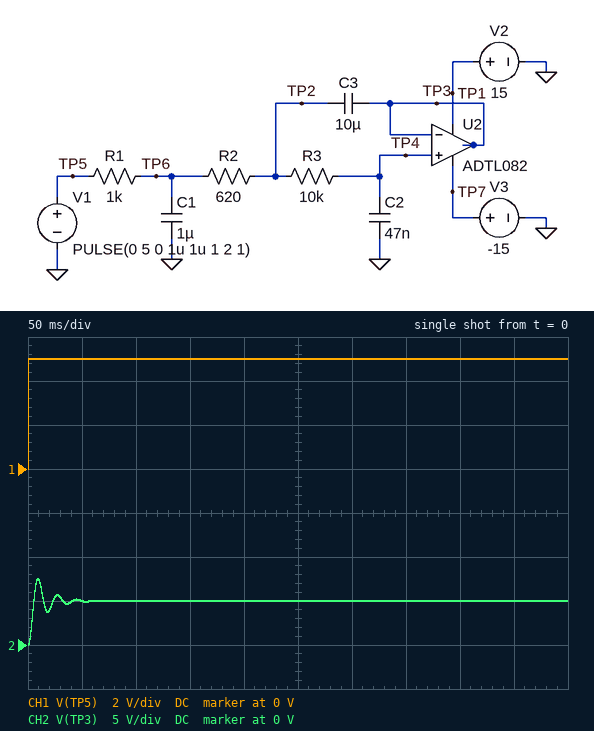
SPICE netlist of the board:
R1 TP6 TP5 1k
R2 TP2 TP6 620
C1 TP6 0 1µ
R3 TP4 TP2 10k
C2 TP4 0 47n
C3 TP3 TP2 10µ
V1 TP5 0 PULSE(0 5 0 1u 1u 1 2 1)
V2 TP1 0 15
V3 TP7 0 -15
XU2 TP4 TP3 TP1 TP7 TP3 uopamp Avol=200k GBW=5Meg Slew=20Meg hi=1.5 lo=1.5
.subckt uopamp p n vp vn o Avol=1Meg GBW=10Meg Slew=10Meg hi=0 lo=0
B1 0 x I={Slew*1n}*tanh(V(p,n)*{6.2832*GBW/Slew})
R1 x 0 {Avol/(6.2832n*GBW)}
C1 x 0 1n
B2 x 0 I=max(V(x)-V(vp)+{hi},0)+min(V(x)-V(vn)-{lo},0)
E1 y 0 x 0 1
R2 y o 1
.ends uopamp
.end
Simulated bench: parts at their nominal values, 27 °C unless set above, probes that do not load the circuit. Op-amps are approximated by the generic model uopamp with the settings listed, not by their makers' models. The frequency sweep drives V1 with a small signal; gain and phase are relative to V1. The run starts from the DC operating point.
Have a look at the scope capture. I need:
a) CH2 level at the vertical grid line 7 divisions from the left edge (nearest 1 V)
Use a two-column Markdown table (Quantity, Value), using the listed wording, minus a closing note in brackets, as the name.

| Quantity | Value |
|---|---|
| CH2 level at the vertical grid line 7 divisions from the left edge | 5 V |
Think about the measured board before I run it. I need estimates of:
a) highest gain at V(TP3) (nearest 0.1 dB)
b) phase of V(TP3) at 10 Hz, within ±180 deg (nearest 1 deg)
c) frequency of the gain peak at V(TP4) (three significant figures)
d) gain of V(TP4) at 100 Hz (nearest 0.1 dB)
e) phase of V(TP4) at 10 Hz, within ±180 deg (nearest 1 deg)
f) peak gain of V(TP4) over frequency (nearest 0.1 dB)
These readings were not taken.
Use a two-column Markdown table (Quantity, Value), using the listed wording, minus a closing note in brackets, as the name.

| Quantity | Value |
|---|---|
| highest gain at V(TP3) | 7.6 dB |
| phase of V(TP3) at 10 Hz, within ±180 deg | -6 deg |
| frequency of the gain peak at V(TP4) | 54.8 Hz |
| gain of V(TP4) at 100 Hz | -6.9 dB |
| phase of V(TP4) at 10 Hz, within ±180 deg | -6 deg |
| peak gain of V(TP4) over frequency | 7.6 dB |
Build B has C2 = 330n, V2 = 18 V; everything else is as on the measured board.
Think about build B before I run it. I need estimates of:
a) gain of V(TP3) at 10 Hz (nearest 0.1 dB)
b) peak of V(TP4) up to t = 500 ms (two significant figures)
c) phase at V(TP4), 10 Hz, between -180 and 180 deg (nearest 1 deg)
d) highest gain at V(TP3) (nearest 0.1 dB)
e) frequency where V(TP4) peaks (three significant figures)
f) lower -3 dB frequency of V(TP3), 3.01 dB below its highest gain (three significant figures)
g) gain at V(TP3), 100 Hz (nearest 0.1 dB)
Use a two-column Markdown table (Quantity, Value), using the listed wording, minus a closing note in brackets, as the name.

| Quantity | Value |
|---|---|
| gain of V(TP3) at 10 Hz | 1.6 dB |
| peak of V(TP4) up to t = 500 ms | 6.9 V |
| phase at V(TP4), 10 Hz, between -180 and 180 deg | -21 deg |
| highest gain at V(TP3) | 4.8 dB |
| frequency where V(TP4) peaks | 19.4 Hz |
| lower -3 dB frequency of V(TP3), 3.01 dB below its highest gain | 10.6 Hz |
| gain at V(TP3), 100 Hz | -26.7 dB |
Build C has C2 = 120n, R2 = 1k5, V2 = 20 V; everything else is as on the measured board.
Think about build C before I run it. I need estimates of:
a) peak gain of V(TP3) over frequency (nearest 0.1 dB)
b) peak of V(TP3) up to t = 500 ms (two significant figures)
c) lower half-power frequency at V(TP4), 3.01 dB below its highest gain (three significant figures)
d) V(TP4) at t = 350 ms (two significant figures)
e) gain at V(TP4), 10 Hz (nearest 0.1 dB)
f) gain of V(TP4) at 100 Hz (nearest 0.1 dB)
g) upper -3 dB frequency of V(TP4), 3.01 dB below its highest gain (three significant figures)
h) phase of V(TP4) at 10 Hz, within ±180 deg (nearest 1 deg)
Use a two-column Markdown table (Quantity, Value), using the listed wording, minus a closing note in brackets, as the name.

| Quantity | Value |
|---|---|
| peak gain of V(TP3) over frequency | 9.3 dB |
| peak of V(TP3) up to t = 500 ms | 7.9 V |
| lower half-power frequency at V(TP4), 3.01 dB below its highest gain | 22.4 Hz |
| V(TP4) at t = 350 ms | 5.0 V |
| gain at V(TP4), 10 Hz | 1.0 dB |
| gain of V(TP4) at 100 Hz | -21.4 dB |
| upper -3 dB frequency of V(TP4), 3.01 dB below its highest gain | 32.7 Hz |
| phase of V(TP4) at 10 Hz, within ±180 deg | -10 deg |
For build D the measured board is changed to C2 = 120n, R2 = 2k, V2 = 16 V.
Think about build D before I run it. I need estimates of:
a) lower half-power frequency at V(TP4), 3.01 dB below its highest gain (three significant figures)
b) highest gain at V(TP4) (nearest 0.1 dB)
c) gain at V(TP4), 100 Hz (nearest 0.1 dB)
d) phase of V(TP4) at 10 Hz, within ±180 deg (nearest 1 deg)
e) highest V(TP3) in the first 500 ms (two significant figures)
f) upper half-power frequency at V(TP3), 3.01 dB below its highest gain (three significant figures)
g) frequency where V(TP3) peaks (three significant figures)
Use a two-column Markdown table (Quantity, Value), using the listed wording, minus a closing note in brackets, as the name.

| Quantity | Value |
|---|---|
| lower half-power frequency at V(TP4), 3.01 dB below its highest gain | 21.1 Hz |
| highest gain at V(TP4) | 10.1 dB |
| gain at V(TP4), 100 Hz | -23.2 dB |
| phase of V(TP4) at 10 Hz, within ±180 deg | -10 deg |
| highest V(TP3) in the first 500 ms | 8.0 V |
| upper half-power frequency at V(TP3), 3.01 dB below its highest gain | 29.7 Hz |
| frequency where V(TP3) peaks | 25.8 Hz |
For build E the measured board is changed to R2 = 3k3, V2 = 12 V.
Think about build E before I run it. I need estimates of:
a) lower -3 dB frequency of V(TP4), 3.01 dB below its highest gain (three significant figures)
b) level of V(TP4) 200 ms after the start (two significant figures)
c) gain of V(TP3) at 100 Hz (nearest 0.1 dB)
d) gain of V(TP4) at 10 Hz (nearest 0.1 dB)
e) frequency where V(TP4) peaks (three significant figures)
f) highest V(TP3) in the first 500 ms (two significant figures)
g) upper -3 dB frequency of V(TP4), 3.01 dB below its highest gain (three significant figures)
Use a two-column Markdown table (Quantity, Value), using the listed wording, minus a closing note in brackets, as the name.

| Quantity | Value |
|---|---|
| lower -3 dB frequency of V(TP4), 3.01 dB below its highest gain | 31.3 Hz |
| level of V(TP4) 200 ms after the start | 4.9 V |
| gain of V(TP3) at 100 Hz | -17.8 dB |
| gain of V(TP4) at 10 Hz | 0.7 dB |
| frequency where V(TP4) peaks | 35.1 Hz |
| highest V(TP3) in the first 500 ms | 8.6 V |
| upper -3 dB frequency of V(TP4), 3.01 dB below its highest gain | 38.5 Hz |
